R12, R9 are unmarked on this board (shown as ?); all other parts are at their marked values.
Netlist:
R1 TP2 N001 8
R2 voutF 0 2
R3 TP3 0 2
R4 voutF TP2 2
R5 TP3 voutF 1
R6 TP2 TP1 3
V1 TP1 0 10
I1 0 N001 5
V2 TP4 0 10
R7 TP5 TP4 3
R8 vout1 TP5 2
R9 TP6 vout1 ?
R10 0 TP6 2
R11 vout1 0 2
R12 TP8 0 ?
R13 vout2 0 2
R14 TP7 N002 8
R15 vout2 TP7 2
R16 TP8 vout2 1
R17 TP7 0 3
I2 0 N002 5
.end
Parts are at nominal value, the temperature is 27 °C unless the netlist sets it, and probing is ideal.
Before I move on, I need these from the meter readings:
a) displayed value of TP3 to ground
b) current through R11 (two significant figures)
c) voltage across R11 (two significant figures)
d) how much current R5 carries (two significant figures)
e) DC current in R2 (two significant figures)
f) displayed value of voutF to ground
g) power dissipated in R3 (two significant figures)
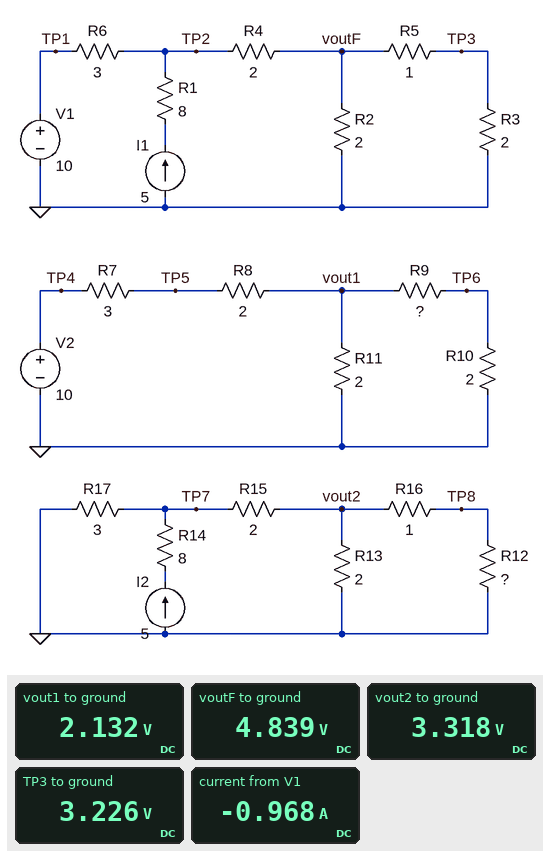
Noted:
3.226 V
1.1 A
2.1 V
1.6 A
2.4 A
4.839 V
5.2 W
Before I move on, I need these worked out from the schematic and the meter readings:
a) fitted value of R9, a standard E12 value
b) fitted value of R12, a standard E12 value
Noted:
2.2 Ω
3.9 Ω
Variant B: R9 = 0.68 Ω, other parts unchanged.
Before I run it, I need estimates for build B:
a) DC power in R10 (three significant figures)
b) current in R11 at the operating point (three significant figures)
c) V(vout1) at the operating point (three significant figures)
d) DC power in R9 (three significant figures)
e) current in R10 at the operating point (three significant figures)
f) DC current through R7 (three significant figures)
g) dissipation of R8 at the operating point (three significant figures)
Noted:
967 mW
932 mA
1.86 V
329 mW
695 mA
1.63 A
5.30 W
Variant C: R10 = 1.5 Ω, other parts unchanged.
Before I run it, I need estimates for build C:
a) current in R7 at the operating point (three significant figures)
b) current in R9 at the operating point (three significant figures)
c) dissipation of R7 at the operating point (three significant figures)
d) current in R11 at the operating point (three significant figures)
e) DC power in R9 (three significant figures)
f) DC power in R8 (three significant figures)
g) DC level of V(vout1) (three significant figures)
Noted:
1.59 A
557 mA
7.56 W
1.03 A
683 mW
5.04 W
2.06 V
